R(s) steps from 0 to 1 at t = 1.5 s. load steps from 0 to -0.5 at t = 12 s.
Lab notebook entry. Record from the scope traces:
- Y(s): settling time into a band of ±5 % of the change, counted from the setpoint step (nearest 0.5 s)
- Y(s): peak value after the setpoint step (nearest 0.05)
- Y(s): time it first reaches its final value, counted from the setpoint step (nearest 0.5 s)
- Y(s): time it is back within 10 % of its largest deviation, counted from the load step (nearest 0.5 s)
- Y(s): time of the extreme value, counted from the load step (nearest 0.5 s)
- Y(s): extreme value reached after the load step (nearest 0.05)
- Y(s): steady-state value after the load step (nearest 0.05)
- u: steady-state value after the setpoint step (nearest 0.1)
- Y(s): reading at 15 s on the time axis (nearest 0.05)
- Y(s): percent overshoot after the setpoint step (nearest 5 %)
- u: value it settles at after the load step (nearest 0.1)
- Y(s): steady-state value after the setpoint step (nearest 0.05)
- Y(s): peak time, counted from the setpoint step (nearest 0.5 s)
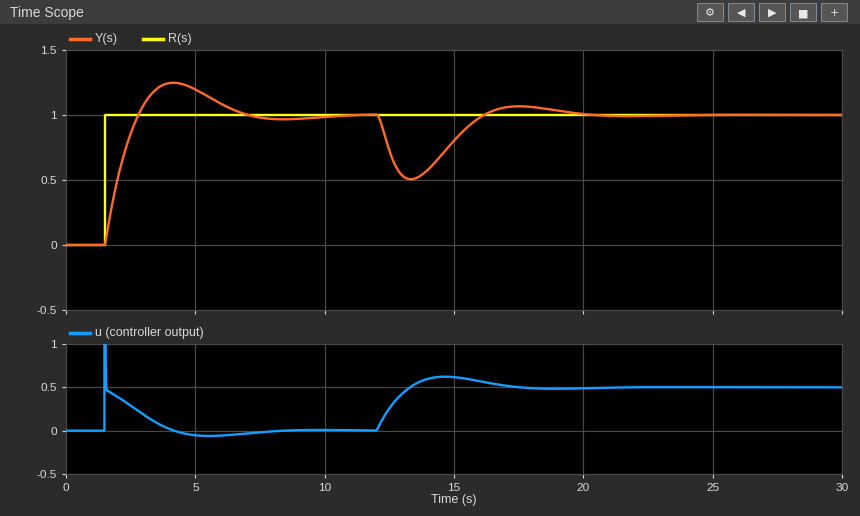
5.0 s
1.25
1.5 s
6.5 s
1.5 s
0.50
1.00
0.0
0.80
25 %
0.5
1.00
2.5 s
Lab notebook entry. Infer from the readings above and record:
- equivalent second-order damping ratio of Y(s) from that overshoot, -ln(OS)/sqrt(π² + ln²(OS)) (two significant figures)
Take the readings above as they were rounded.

0.40
